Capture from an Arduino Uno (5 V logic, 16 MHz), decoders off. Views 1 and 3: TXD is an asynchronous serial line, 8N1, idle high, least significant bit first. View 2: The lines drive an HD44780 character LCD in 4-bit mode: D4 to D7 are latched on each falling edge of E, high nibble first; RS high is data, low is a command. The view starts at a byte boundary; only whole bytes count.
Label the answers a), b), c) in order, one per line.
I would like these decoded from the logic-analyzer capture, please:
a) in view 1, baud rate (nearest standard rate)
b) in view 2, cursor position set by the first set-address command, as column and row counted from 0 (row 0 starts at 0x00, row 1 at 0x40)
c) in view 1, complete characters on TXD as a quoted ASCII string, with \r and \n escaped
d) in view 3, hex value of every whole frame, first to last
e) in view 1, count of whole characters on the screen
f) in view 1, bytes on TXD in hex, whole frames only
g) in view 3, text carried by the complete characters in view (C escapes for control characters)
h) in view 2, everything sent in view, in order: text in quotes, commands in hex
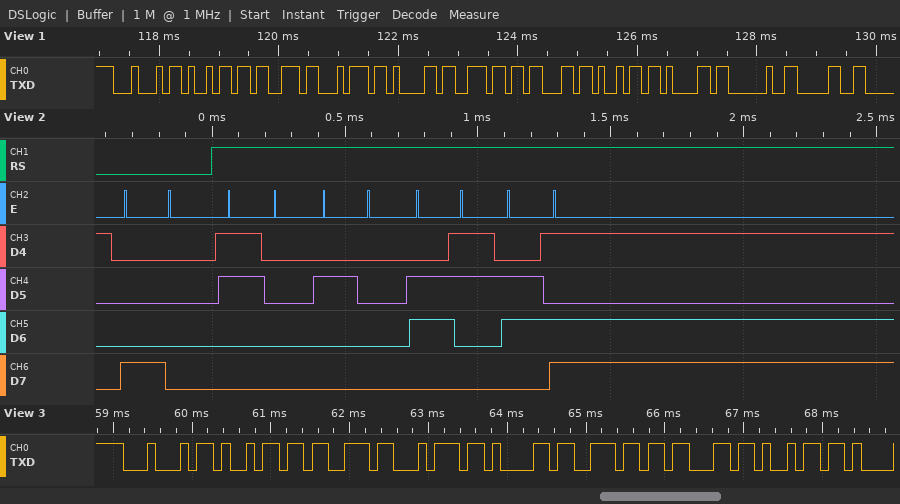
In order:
a) 9600 baud
b) column 0, row 0
c) "Distancia 0"
d) 44 69 73 74 61 6E 63 69
e) 11
f) 44 69 73 74 61 6E 63 69 61 20 30
g) "Distanci"
h) 0x80 "0 cm"
